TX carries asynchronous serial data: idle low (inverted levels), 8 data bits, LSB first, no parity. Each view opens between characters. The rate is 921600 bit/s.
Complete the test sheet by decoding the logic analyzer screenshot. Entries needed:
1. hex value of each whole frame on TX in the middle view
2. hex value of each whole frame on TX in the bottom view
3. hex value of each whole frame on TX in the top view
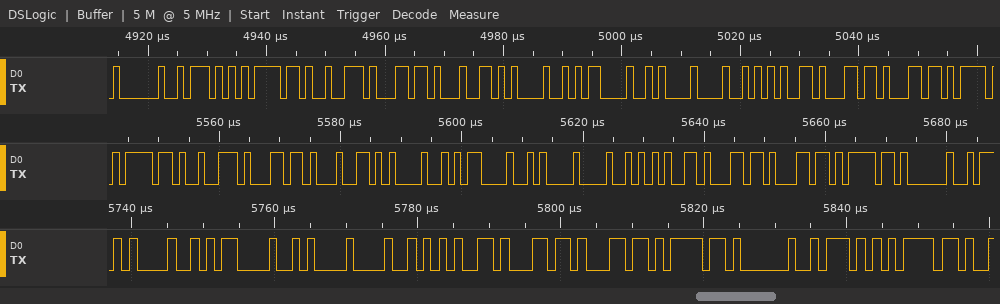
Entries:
21, 1B, 27, 37, BD, E5, EB, 6F, 35, 27, 27, 21, BF
BD, E5, EB, 6F, 35, 27, 27, 21, BF, 51, 21
BF, 51, 21, 1B, 27, 37, BD, E5, EB, 6F, 35, 27, 27
